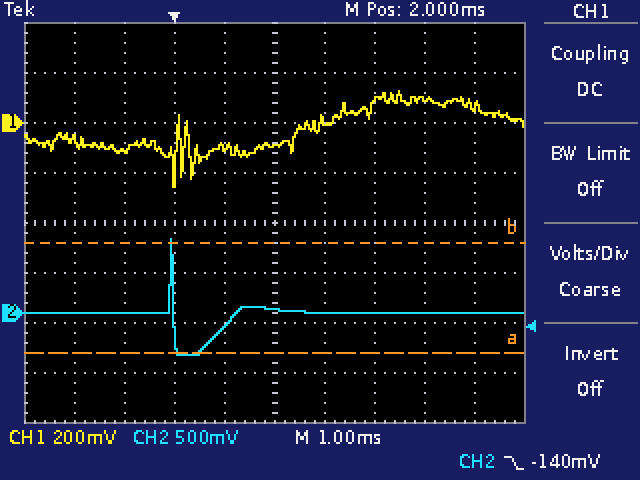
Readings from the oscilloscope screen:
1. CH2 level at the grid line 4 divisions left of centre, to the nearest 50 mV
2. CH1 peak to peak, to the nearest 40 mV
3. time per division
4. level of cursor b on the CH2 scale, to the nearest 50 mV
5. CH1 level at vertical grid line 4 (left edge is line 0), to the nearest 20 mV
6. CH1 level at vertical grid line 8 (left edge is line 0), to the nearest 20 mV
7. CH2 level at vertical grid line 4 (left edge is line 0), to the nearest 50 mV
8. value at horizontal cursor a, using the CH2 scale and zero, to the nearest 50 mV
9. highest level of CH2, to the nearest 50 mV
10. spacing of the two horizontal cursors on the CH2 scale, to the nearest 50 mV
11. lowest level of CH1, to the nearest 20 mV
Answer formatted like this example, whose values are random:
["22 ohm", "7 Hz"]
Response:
["0 mV", "400 mV", "1 ms", "700 mV", "-100 mV", "100 mV", "-150 mV", "-400 mV", "750 mV", "1.10 V", "-260 mV"]
